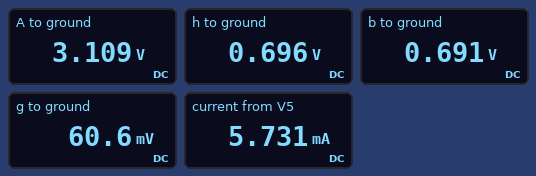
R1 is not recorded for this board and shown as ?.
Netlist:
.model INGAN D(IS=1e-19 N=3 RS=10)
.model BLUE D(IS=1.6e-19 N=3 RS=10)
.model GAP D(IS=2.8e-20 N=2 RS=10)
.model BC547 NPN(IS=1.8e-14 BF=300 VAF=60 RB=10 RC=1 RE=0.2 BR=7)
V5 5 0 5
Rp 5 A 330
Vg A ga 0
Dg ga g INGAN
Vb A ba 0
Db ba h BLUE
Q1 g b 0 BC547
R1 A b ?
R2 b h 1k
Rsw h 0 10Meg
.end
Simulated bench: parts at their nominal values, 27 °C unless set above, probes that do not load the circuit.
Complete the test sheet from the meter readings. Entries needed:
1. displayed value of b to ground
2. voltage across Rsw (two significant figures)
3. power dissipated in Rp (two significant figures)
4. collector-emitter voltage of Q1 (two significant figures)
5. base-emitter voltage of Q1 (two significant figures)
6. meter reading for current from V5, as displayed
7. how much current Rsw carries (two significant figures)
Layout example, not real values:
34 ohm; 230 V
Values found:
0.691 V; 700 mV; 11 mW; 61 mV; 690 mV; 5.731 mA; 70 nA
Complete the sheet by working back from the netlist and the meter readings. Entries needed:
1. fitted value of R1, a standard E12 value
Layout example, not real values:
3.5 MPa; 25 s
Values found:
18 kΩ
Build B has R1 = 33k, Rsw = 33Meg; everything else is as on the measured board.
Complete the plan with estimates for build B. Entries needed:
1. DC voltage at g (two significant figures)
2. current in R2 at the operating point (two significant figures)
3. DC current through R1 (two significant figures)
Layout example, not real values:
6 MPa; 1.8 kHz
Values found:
76 mV; 6.3 µA; 74 µA
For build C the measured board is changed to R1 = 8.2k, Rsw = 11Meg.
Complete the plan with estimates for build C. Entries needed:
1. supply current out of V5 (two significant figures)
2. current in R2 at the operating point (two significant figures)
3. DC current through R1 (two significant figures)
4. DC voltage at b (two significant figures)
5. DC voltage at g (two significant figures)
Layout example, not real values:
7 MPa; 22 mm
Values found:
5.8 mA; 3.7 µA; 290 µA; 700 mV; 43 mV
